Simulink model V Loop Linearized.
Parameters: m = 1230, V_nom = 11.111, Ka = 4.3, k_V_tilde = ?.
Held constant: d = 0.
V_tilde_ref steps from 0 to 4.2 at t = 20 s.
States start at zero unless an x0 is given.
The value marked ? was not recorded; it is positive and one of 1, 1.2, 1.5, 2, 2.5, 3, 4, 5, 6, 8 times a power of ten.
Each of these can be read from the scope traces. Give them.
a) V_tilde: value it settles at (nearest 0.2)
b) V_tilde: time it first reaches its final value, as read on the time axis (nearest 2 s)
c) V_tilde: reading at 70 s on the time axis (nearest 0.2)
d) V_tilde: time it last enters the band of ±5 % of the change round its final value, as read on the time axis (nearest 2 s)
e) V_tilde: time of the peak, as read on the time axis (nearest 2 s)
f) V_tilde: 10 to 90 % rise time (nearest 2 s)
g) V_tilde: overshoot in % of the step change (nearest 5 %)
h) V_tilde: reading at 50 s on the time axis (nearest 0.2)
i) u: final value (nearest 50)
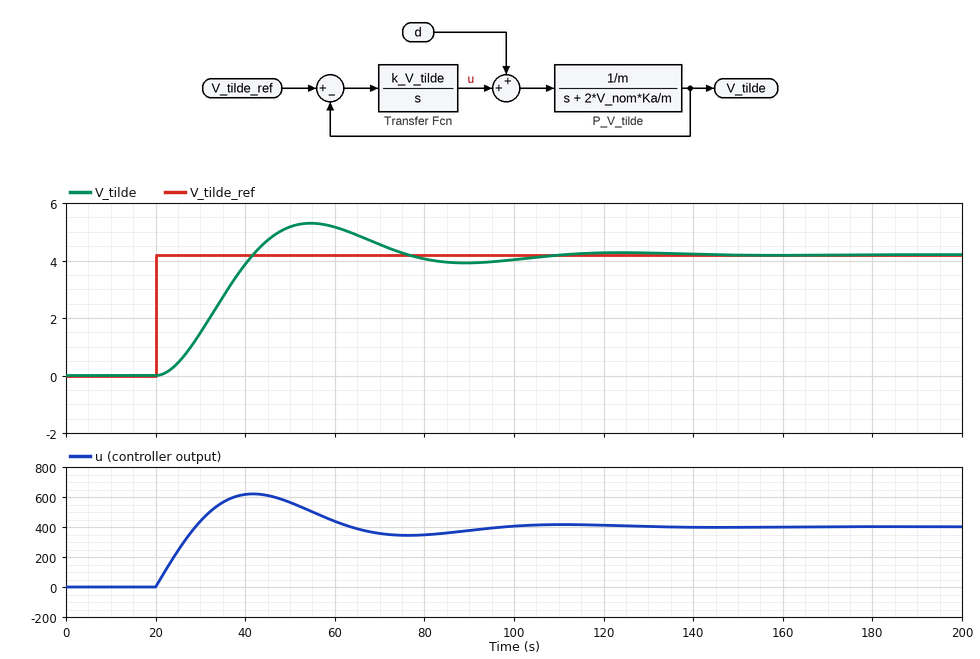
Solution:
4.2
42 s
4.6
98 s
54 s
14 s
25 %
5.2
400
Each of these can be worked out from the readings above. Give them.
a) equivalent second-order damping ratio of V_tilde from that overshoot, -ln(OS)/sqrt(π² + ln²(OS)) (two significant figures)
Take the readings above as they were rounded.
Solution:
0.40
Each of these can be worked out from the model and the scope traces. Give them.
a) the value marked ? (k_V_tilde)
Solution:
12
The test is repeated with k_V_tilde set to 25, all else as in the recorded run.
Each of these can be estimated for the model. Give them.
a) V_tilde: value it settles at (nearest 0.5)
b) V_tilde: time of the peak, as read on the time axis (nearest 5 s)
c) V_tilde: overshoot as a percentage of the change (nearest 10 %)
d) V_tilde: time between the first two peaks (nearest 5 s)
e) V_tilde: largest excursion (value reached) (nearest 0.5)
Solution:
4.0
45 s
40 %
45 s
6.0
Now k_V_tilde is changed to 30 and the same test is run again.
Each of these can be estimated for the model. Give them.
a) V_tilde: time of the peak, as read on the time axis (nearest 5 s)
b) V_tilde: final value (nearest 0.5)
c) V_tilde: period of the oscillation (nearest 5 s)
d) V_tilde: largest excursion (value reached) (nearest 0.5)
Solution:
40 s
4.0
40 s
6.0
